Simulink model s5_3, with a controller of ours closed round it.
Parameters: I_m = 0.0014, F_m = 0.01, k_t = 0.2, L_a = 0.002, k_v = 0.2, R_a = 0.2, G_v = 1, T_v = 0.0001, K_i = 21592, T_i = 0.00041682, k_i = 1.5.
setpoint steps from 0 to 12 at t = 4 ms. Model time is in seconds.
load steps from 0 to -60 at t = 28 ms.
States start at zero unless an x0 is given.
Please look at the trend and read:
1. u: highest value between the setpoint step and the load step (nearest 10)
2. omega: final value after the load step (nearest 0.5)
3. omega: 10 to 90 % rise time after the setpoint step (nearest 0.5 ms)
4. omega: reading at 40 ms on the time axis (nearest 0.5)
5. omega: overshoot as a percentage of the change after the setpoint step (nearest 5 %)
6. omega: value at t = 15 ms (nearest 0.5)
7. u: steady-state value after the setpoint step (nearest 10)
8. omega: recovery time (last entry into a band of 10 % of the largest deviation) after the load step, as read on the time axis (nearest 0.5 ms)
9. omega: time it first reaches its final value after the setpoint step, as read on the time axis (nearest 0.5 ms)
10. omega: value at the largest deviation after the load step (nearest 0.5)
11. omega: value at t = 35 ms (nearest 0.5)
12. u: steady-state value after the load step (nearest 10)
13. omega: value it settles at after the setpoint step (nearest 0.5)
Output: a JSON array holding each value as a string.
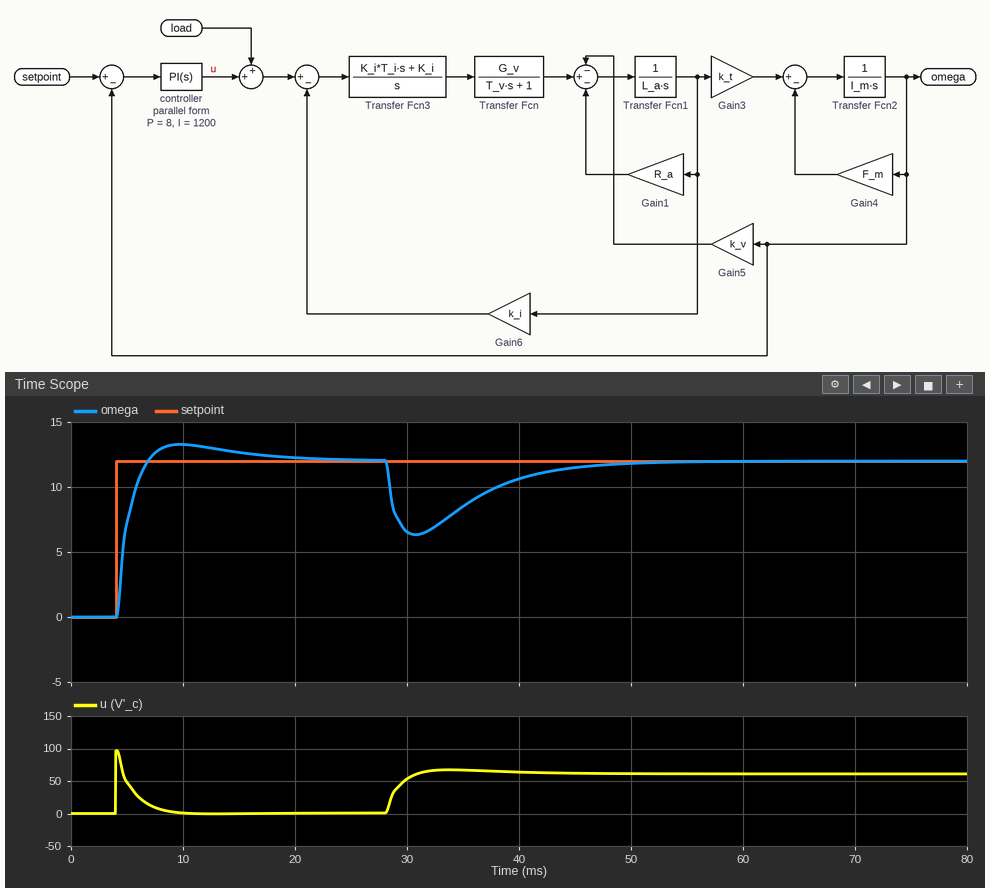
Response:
["100", "12.0", "2.0 ms", "10.5", "10 %", "12.5", "0", "44.5 ms", "7.0 ms", "6.5", "8.5", "60", "12.0"]
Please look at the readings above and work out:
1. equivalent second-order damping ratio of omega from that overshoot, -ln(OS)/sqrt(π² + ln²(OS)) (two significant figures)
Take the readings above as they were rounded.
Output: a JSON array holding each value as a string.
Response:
["0.59"]
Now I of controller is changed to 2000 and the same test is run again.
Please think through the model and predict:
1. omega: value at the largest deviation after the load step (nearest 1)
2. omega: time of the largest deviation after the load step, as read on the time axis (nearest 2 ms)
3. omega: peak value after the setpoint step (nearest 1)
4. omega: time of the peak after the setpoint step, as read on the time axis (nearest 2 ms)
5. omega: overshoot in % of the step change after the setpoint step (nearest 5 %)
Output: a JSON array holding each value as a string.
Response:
["7", "30 ms", "14", "8 ms", "15 %"]
